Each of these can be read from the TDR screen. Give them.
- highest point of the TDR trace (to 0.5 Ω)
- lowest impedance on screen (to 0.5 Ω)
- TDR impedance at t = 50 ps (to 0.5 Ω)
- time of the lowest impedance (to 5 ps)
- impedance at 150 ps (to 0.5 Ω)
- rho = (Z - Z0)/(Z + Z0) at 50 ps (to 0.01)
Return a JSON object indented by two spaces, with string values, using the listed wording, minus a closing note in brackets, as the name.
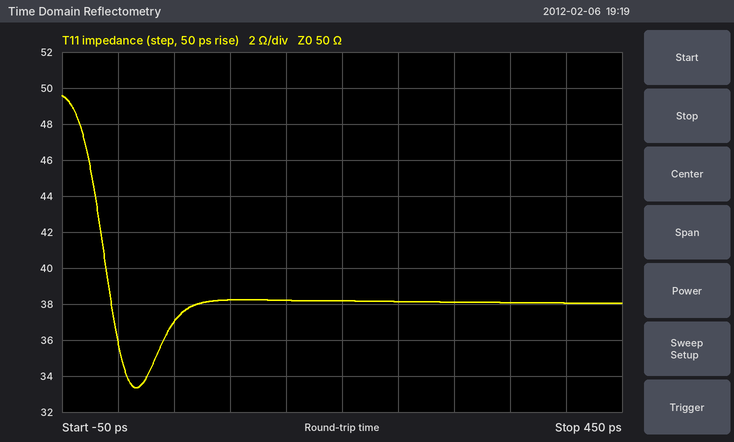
{
  "highest point of the TDR trace": "49.5 Ω",
  "lowest impedance on screen": "33.5 Ω",
  "TDR impedance at t = 50 ps": "37.0 Ω",
  "time of the lowest impedance": "15 ps",
  "impedance at 150 ps": "38.0 Ω",
  "rho = (Z - Z0)/(Z + Z0) at 50 ps": "-0.15"
}
